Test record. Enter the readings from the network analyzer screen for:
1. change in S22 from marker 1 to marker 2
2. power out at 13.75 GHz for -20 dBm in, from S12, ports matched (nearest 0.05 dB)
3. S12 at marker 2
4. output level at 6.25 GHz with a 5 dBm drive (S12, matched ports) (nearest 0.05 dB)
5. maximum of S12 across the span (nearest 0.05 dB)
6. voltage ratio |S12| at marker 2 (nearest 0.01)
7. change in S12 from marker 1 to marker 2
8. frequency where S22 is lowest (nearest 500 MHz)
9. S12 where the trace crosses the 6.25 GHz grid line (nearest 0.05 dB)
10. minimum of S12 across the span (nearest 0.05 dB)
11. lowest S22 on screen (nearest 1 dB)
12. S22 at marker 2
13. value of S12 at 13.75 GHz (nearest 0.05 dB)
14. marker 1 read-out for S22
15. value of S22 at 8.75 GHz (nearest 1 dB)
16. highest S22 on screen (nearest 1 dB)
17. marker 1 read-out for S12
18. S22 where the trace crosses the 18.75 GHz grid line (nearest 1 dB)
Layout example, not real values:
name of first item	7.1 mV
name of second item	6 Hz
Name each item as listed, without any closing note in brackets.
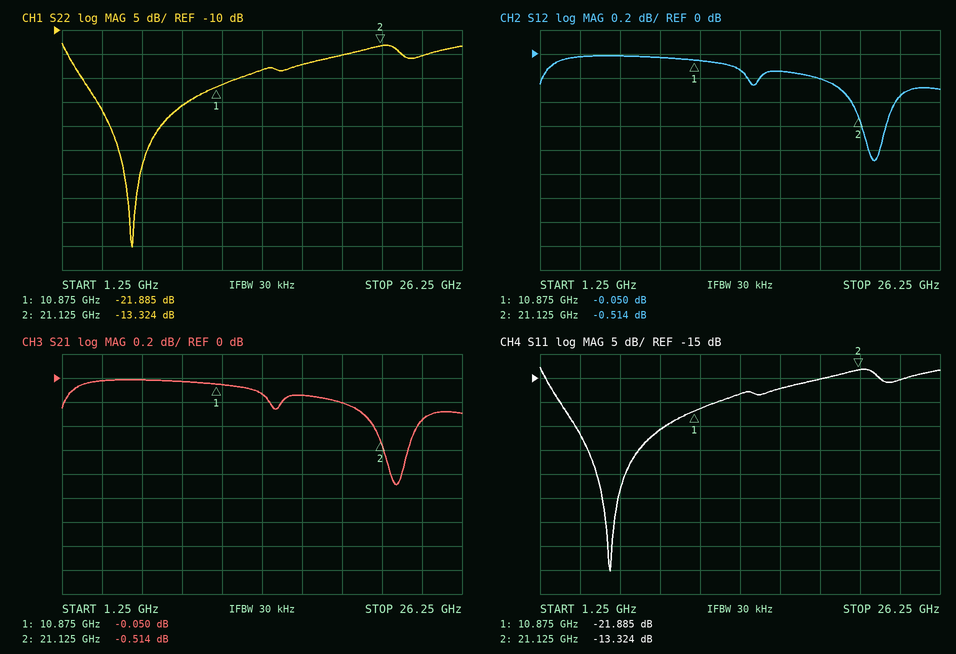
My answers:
change in S22 from marker 1 to marker 2	8.561 dB
power out at 13.75 GHz for -20 dBm in, from S12, ports matched	-20.15 dBm
S12 at marker 2	-0.514 dB
output level at 6.25 GHz with a 5 dBm drive (S12, matched ports)	5.00 dBm
maximum of S12 across the span	0.00 dB
voltage ratio |S12| at marker 2	0.94
change in S12 from marker 1 to marker 2	-0.464 dB
frequency where S22 is lowest	5.5 GHz
S12 where the trace crosses the 6.25 GHz grid line	0.00 dB
minimum of S12 across the span	-0.90 dB
lowest S22 on screen	-55 dB
S22 at marker 2	-13.324 dB
value of S12 at 13.75 GHz	-0.15 dB
marker 1 read-out for S22	-21.885 dB
value of S22 at 8.75 GHz	-26 dB
highest S22 on screen	-13 dB
marker 1 read-out for S12	-0.050 dB
S22 where the trace crosses the 18.75 GHz grid line	-15 dB
